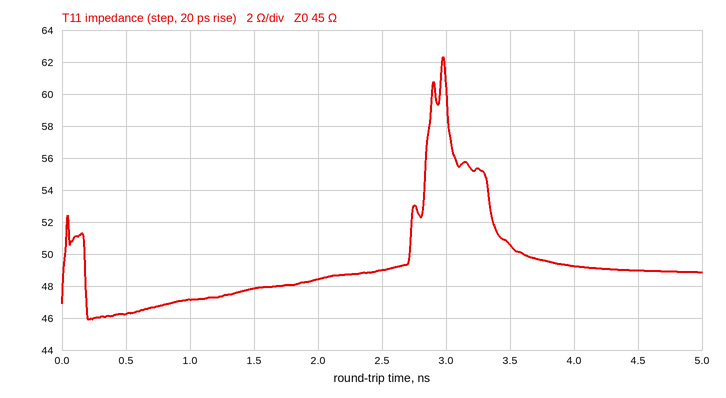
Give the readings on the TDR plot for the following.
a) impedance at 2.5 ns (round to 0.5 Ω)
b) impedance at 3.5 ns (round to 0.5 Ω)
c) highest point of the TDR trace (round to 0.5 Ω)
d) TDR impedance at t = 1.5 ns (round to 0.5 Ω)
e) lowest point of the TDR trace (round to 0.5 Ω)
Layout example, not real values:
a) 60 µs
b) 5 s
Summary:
a) 49.0 Ω
b) 50.5 Ω
c) 62.5 Ω
d) 48.0 Ω
e) 46.0 Ω
